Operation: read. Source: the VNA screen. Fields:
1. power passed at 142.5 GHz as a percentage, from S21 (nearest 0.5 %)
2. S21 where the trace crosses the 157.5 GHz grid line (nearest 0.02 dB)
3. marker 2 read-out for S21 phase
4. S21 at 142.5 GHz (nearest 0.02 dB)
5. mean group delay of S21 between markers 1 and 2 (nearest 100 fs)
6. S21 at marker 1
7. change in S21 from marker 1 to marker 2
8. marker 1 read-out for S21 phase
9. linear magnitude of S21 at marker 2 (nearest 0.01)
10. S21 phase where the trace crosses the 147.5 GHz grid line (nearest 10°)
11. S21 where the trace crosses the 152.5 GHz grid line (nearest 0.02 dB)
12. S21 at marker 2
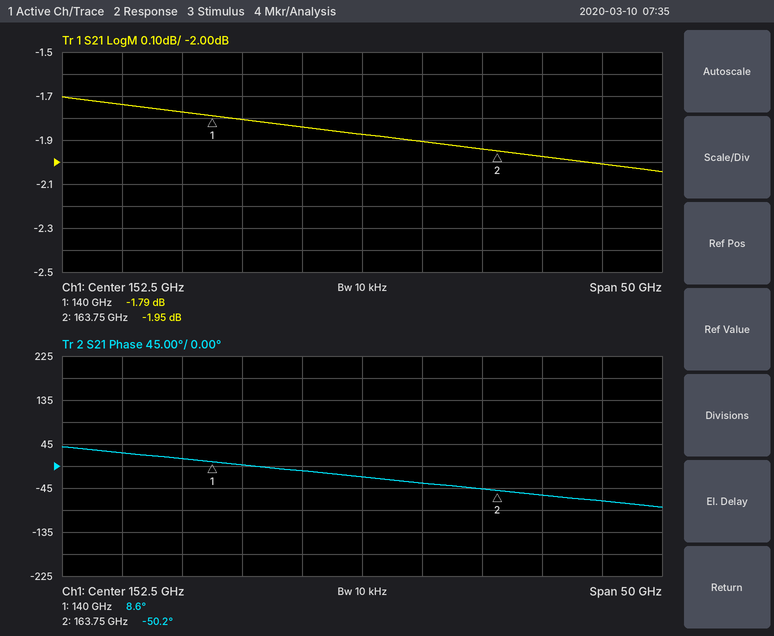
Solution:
66.0 %
-1.90 dB
-50.2°
-1.80 dB
6.9 ps
-1.79 dB
-0.16 dB
8.6°
0.80
-10°
-1.88 dB
-1.95 dB
